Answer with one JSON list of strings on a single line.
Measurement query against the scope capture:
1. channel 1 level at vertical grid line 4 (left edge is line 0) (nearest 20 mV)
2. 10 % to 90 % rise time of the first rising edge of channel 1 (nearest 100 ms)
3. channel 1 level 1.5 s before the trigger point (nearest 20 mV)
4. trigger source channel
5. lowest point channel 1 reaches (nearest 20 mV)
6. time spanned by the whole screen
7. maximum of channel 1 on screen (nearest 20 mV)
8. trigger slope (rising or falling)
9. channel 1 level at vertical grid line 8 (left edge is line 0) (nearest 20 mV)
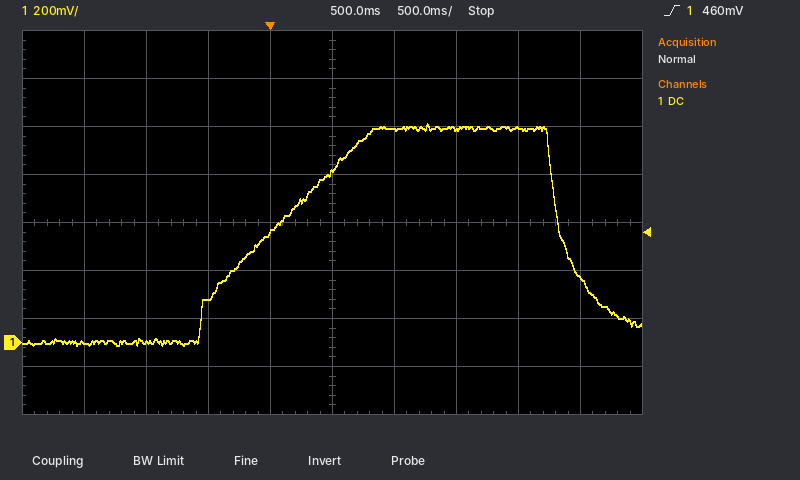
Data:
["460 mV", "1.2 s", "0 mV", "channel 1", "-20 mV", "5 s", "920 mV", "rising", "900 mV"]
